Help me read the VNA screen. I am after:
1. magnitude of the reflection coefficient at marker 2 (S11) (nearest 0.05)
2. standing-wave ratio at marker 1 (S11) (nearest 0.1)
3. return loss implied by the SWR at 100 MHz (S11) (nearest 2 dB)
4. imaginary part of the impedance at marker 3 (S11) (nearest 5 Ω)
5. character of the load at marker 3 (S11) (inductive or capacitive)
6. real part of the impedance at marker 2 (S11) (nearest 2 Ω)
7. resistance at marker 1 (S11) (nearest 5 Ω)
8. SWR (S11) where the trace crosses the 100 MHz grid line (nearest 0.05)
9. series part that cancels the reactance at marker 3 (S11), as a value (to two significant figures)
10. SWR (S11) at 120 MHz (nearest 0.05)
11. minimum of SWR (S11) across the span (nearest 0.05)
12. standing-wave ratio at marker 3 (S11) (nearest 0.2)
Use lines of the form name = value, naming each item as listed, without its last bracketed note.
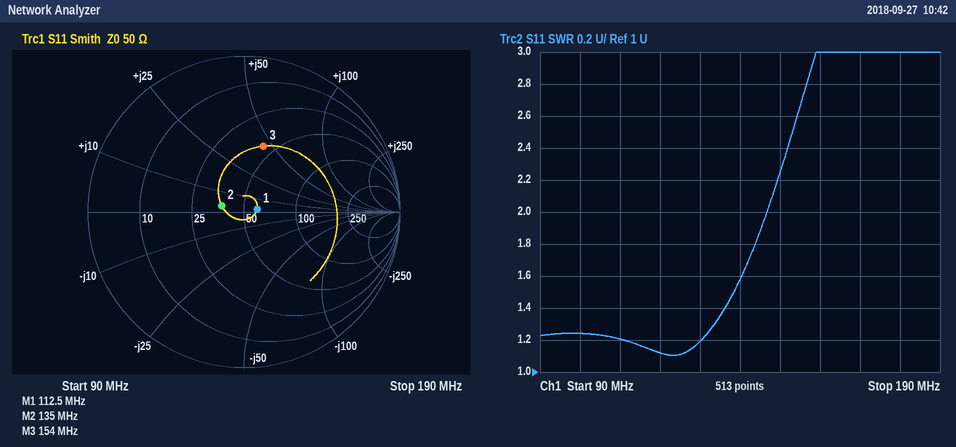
magnitude of the reflection coefficient at marker 2 (S11) = 0.15
standing-wave ratio at marker 1 (S11) = 1.2
return loss implied by the SWR at 100 MHz (S11) = 20 dB
imaginary part of the impedance at marker 3 (S11) = +45 Ω
character of the load at marker 3 (S11) = inductive
real part of the impedance at marker 2 (S11) = 38 Ω
resistance at marker 1 (S11) = 60 Ω
SWR (S11) where the trace crosses the 100 MHz grid line = 1.25
series part that cancels the reactance at marker 3 (S11), as a value = 23 pF
SWR (S11) at 120 MHz = 1.10
minimum of SWR (S11) across the span = 1.10
standing-wave ratio at marker 3 (S11) = 2.6
